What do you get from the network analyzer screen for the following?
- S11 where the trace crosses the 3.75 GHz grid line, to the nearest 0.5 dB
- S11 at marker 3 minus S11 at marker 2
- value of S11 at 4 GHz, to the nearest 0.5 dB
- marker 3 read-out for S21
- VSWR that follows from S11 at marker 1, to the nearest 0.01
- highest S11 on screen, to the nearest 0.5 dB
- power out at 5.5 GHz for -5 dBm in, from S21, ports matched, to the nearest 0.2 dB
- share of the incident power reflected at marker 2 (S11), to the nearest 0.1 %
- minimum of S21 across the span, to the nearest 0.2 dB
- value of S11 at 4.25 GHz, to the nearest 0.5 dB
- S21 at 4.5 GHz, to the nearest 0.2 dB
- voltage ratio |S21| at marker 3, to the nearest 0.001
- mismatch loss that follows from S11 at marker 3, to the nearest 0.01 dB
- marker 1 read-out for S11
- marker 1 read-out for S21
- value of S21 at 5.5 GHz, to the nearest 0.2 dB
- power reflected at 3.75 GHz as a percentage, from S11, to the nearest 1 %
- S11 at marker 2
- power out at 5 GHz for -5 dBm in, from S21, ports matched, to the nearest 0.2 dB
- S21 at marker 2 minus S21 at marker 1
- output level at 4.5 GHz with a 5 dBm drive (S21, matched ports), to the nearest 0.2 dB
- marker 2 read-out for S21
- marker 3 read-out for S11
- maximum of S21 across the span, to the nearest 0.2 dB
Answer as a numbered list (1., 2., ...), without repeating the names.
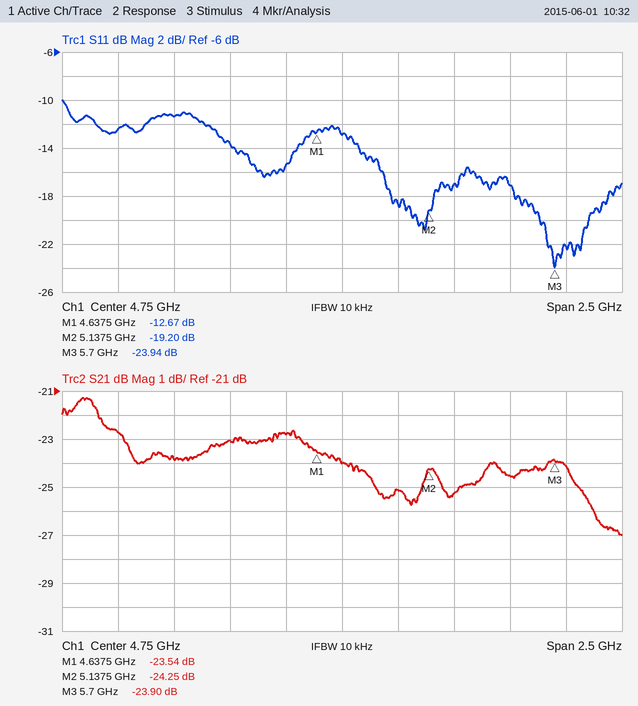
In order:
1. -12.5 dB
2. -4.74 dB
3. -11.5 dB
4. -23.90 dB
5. 1.61
6. -10.0 dB
7. -29.6 dBm
8. 1.2 %
9. -27.0 dB
10. -13.5 dB
11. -22.8 dB
12. 0.064
13. 0.02 dB
14. -12.67 dB
15. -23.54 dB
16. -24.6 dB
17. 6 %
18. -19.20 dB
19. -30.2 dBm
20. -0.71 dB
21. -17.8 dBm
22. -24.25 dB
23. -23.94 dB
24. -21.2 dB
